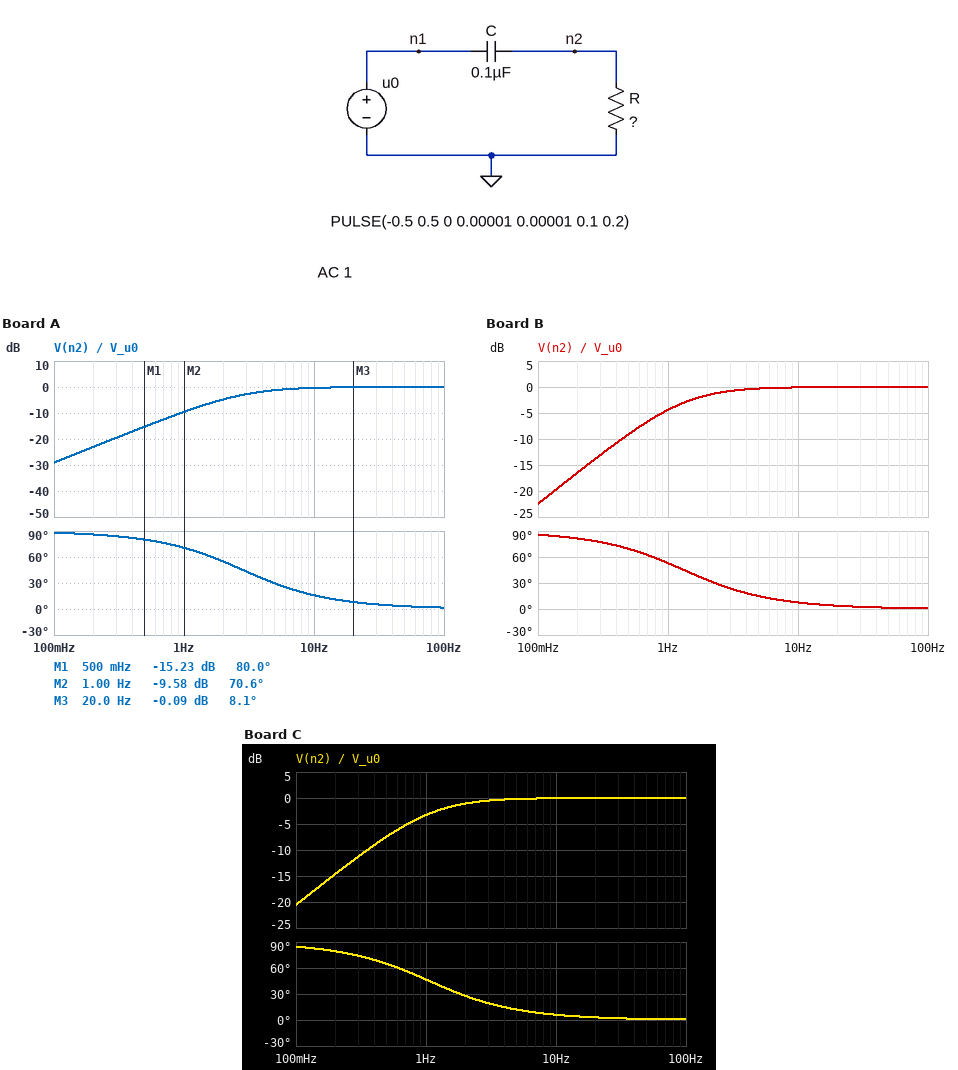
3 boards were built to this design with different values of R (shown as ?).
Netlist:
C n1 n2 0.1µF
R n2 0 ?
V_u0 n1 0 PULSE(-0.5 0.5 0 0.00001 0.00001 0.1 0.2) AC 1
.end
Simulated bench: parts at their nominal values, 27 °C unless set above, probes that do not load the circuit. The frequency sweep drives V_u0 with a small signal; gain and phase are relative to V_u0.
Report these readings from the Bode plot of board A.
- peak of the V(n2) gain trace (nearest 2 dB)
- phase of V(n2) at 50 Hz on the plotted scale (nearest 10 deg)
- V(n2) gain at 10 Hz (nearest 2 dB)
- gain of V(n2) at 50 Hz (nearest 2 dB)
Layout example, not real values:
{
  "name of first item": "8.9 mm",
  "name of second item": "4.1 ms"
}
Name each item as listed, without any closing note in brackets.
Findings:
{
  "peak of the V(n2) gain trace": "0 dB",
  "phase of V(n2) at 50 Hz on the plotted scale": "0 deg",
  "V(n2) gain at 10 Hz": "0 dB",
  "gain of V(n2) at 50 Hz": "0 dB"
}
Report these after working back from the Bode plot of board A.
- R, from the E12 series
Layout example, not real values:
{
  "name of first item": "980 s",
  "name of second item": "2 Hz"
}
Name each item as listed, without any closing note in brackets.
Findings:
{
  "R, from the E12 series": "560 kΩ"
}
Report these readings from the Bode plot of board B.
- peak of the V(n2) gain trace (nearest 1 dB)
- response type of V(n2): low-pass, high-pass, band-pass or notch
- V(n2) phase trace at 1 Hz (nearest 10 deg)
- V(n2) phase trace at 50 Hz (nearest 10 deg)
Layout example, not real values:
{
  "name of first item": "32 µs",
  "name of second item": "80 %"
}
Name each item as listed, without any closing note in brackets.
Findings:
{
  "peak of the V(n2) gain trace": "0 dB",
  "response type of V(n2): low-pass, high-pass, band-pass or notch": "high-pass",
  "V(n2) phase trace at 1 Hz": "50 deg",
  "V(n2) phase trace at 50 Hz": "0 deg"
}
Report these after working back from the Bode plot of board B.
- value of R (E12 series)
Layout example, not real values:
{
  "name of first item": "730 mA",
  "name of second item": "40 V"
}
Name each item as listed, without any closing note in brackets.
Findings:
{
  "value of R": "1.2 MΩ"
}
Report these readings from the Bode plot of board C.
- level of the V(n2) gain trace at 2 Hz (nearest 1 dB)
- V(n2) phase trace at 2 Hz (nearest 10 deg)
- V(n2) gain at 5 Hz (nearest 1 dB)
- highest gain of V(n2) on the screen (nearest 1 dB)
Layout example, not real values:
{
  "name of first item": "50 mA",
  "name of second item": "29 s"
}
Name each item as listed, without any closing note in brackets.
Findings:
{
  "level of the V(n2) gain trace at 2 Hz": "-1 dB",
  "V(n2) phase trace at 2 Hz": "30 deg",
  "V(n2) gain at 5 Hz": "0 dB",
  "highest gain of V(n2) on the screen": "0 dB"
}
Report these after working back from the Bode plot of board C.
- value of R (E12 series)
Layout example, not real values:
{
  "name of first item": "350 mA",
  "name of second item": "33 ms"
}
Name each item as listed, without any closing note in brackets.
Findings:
{
  "value of R": "1.5 MΩ"
}
